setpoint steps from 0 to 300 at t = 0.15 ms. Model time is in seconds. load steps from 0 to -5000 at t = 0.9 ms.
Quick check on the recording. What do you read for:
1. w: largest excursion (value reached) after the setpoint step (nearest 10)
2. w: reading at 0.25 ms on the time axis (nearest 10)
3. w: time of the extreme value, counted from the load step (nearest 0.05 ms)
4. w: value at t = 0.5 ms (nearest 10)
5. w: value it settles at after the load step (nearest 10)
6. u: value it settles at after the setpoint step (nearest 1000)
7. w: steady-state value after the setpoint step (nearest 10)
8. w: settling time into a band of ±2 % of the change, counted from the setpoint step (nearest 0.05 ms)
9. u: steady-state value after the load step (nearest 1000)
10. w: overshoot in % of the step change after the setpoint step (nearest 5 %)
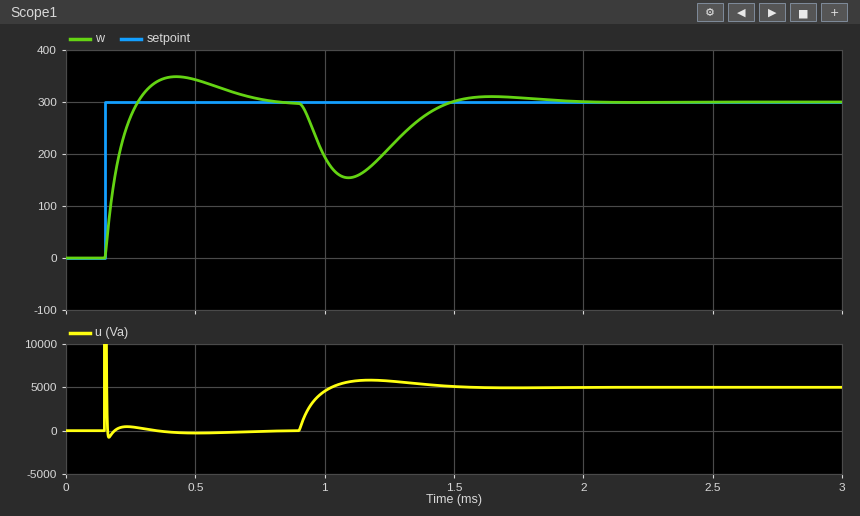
350
270
0.20 ms
340
300
0
300
0.60 ms
5000
15 %
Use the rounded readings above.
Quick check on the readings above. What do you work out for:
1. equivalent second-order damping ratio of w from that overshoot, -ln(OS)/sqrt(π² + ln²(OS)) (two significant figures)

0.52
